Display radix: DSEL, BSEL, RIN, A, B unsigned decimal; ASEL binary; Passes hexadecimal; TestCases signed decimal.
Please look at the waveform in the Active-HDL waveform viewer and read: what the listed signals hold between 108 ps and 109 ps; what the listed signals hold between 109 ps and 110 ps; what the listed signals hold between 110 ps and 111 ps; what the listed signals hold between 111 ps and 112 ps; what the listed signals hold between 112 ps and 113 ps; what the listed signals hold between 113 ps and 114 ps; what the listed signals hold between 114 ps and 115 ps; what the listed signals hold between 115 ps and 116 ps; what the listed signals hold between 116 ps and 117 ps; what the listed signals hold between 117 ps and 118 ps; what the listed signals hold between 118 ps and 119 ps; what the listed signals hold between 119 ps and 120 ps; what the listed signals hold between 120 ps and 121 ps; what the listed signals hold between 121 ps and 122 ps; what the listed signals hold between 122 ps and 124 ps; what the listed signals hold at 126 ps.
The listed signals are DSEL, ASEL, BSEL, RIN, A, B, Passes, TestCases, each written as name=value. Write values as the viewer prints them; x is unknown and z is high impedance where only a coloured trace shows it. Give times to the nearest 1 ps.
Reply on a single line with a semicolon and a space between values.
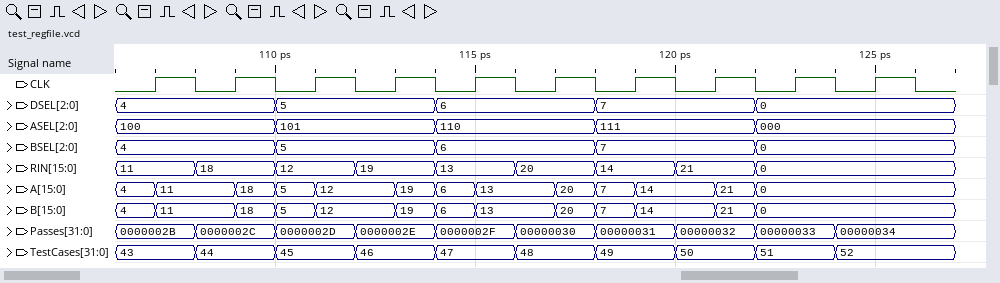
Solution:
DSEL=4, ASEL=100, BSEL=4, RIN=18, A=11, B=11, Passes=0000002C, TestCases=44; DSEL=4, ASEL=100, BSEL=4, RIN=18, A=18, B=18, Passes=0000002C, TestCases=44; DSEL=5, ASEL=101, BSEL=5, RIN=12, A=5, B=5, Passes=0000002D, TestCases=45; DSEL=5, ASEL=101, BSEL=5, RIN=12, A=12, B=12, Passes=0000002D, TestCases=45; DSEL=5, ASEL=101, BSEL=5, RIN=19, A=12, B=12, Passes=0000002E, TestCases=46; DSEL=5, ASEL=101, BSEL=5, RIN=19, A=19, B=19, Passes=0000002E, TestCases=46; DSEL=6, ASEL=110, BSEL=6, RIN=13, A=6, B=6, Passes=0000002F, TestCases=47; DSEL=6, ASEL=110, BSEL=6, RIN=13, A=13, B=13, Passes=0000002F, TestCases=47; DSEL=6, ASEL=110, BSEL=6, RIN=20, A=13, B=13, Passes=00000030, TestCases=48; DSEL=6, ASEL=110, BSEL=6, RIN=20, A=20, B=20, Passes=00000030, TestCases=48; DSEL=7, ASEL=111, BSEL=7, RIN=14, A=7, B=7, Passes=00000031, TestCases=49; DSEL=7, ASEL=111, BSEL=7, RIN=14, A=14, B=14, Passes=00000031, TestCases=49; DSEL=7, ASEL=111, BSEL=7, RIN=21, A=14, B=14, Passes=00000032, TestCases=50; DSEL=7, ASEL=111, BSEL=7, RIN=21, A=21, B=21, Passes=00000032, TestCases=50; DSEL=0, ASEL=000, BSEL=0, RIN=0, A=0, B=0, Passes=00000033, TestCases=51; DSEL=0, ASEL=000, BSEL=0, RIN=0, A=0, B=0, Passes=00000034, TestCases=52
